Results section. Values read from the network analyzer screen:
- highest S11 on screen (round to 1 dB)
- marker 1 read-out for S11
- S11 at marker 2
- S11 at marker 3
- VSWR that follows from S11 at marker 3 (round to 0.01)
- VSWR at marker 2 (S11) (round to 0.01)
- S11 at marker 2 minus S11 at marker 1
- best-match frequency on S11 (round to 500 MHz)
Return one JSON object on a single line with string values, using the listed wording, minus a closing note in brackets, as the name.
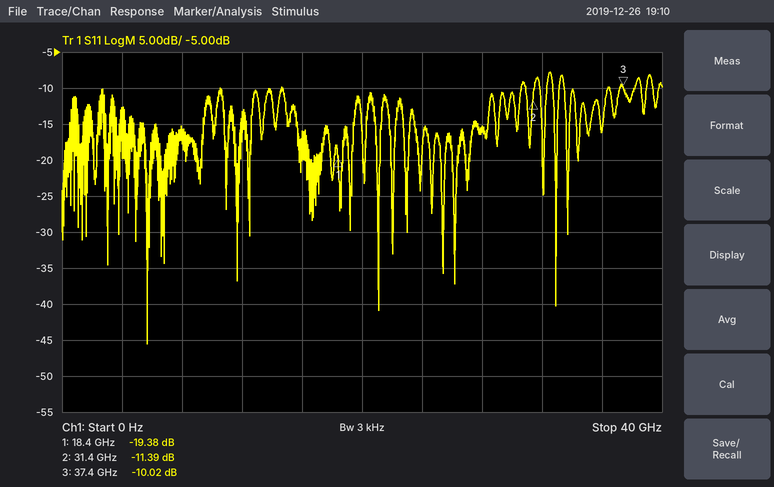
{"highest S11 on screen": "-8 dB", "marker 1 read-out for S11": "-19.38 dB", "S11 at marker 2": "-11.39 dB", "S11 at marker 3": "-10.02 dB", "VSWR that follows from S11 at marker 3": "1.92", "VSWR at marker 2 (S11)": "1.74", "S11 at marker 2 minus S11 at marker 1": "7.99 dB", "best-match frequency on S11": "5.5 GHz"}
